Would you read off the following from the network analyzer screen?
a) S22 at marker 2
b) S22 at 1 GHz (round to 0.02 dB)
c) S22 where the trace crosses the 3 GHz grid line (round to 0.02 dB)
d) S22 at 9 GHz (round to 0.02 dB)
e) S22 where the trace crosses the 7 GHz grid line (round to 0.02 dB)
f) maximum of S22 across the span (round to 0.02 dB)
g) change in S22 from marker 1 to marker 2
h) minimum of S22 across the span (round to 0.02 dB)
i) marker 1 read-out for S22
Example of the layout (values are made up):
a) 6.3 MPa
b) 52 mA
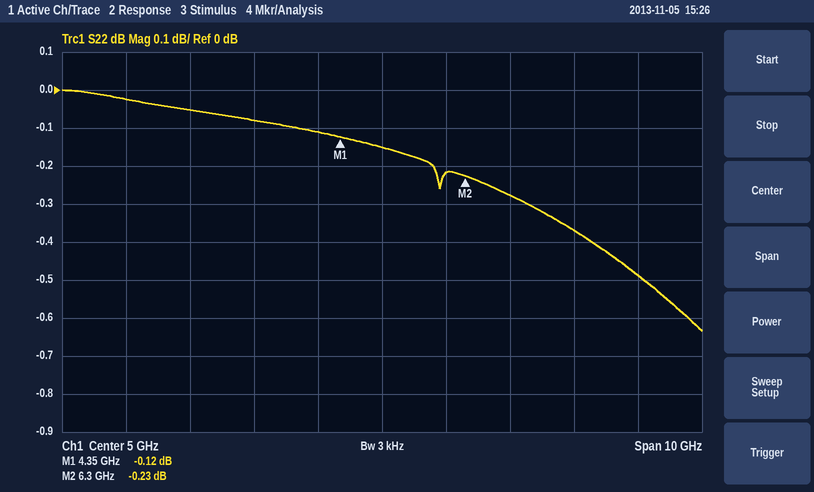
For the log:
a) -0.23 dB
b) -0.02 dB
c) -0.08 dB
d) -0.48 dB
e) -0.28 dB
f) 0.00 dB
g) -0.11 dB
h) -0.64 dB
i) -0.12 dB
